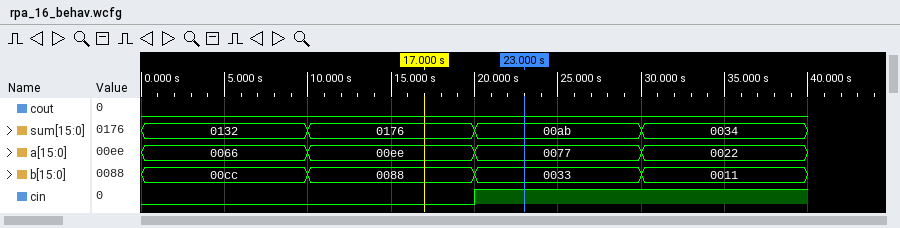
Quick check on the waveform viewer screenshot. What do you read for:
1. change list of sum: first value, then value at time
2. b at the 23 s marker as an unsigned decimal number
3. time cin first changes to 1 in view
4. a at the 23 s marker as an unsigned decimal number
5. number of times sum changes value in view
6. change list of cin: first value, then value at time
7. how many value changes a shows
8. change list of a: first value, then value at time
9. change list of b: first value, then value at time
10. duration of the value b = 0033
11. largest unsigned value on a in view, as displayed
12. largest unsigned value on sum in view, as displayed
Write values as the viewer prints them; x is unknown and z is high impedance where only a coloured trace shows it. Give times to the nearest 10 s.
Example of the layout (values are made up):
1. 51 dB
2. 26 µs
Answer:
1. 0132, 0176 at 10 s, 00ab at 20 s, 0034 at 30 s
2. 51
3. 20 s
4. 119
5. 3
6. 0, 1 at 20 s
7. 3
8. 0066, 00ee at 10 s, 0077 at 20 s, 0022 at 30 s
9. 00cc, 0088 at 10 s, 0033 at 20 s, 0011 at 30 s
10. 10 s
11. 00ee
12. 0176
